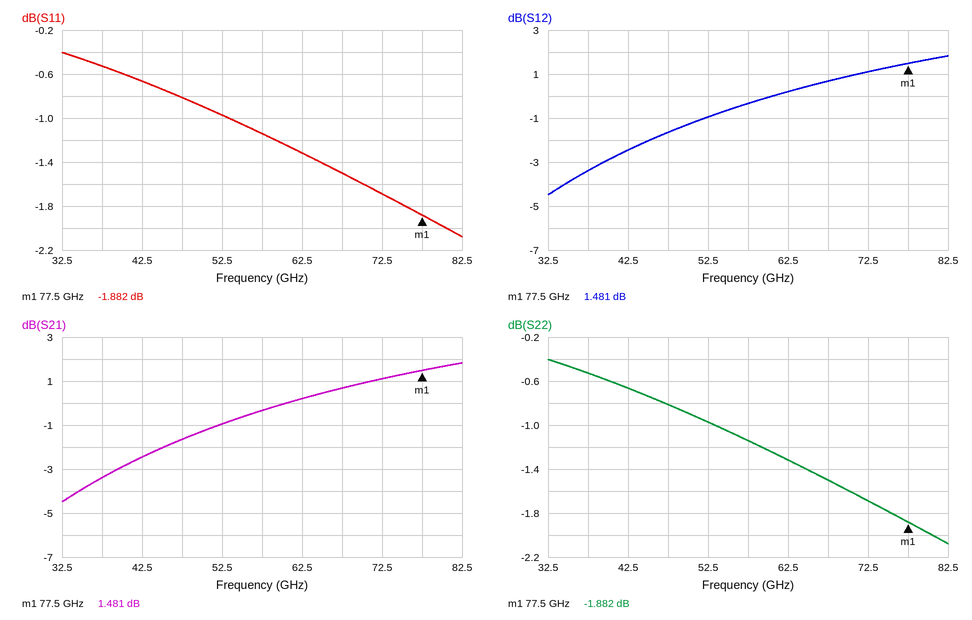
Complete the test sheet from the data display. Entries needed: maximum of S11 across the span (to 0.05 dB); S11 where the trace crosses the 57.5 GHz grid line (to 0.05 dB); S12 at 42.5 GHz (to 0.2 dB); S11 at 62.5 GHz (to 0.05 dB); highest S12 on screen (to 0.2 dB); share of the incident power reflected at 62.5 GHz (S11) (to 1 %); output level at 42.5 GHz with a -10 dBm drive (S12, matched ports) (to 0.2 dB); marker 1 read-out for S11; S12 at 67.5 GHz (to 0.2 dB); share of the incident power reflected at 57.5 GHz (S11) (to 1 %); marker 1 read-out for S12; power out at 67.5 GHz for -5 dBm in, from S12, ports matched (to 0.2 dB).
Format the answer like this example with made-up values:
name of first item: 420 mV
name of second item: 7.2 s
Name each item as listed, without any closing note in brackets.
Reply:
maximum of S11 across the span: -0.40 dB
S11 where the trace crosses the 57.5 GHz grid line: -1.15 dB
S12 at 42.5 GHz: -2.4 dB
S11 at 62.5 GHz: -1.30 dB
highest S12 on screen: 1.8 dB
share of the incident power reflected at 62.5 GHz (S11): 74 %
output level at 42.5 GHz with a -10 dBm drive (S12, matched ports): -12.4 dBm
marker 1 read-out for S11: -1.882 dB
S12 at 67.5 GHz: 0.6 dB
share of the incident power reflected at 57.5 GHz (S11): 77 %
marker 1 read-out for S12: 1.481 dB
power out at 67.5 GHz for -5 dBm in, from S12, ports matched: -4.4 dBm
